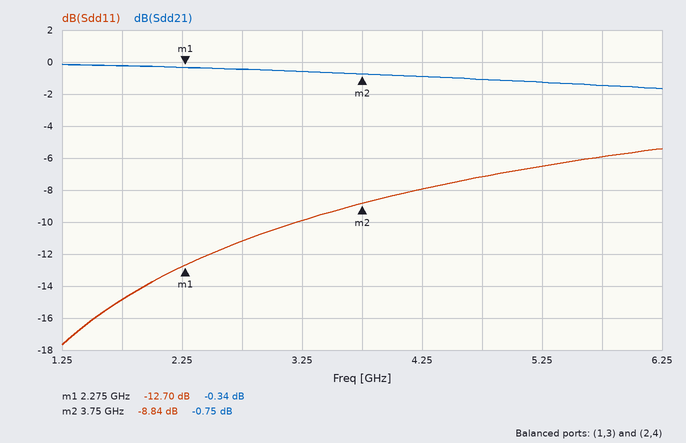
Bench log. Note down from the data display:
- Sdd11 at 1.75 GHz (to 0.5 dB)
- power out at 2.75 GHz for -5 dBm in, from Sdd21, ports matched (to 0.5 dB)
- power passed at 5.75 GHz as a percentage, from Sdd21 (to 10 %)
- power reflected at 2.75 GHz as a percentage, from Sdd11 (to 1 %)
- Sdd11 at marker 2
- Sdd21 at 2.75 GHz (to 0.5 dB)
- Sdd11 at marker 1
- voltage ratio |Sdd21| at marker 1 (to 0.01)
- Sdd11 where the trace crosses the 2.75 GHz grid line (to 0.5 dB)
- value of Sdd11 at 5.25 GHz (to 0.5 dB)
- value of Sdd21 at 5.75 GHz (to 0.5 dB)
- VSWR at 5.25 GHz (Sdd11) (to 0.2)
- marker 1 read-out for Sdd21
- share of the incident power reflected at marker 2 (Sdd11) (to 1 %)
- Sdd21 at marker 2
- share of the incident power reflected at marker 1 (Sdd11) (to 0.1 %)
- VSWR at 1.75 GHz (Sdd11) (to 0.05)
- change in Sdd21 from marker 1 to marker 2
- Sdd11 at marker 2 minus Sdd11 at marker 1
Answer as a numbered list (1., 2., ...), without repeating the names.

1. -15.0 dB
2. -5.5 dBm
3. 70 %
4. 8 %
5. -8.84 dB
6. -0.5 dB
7. -12.70 dB
8. 0.96
9. -11.0 dB
10. -6.5 dB
11. -1.5 dB
12. 2.8
13. -0.34 dB
14. 13 %
15. -0.75 dB
16. 5.4 %
17. 1.45
18. -0.41 dB
19. 3.86 dB
